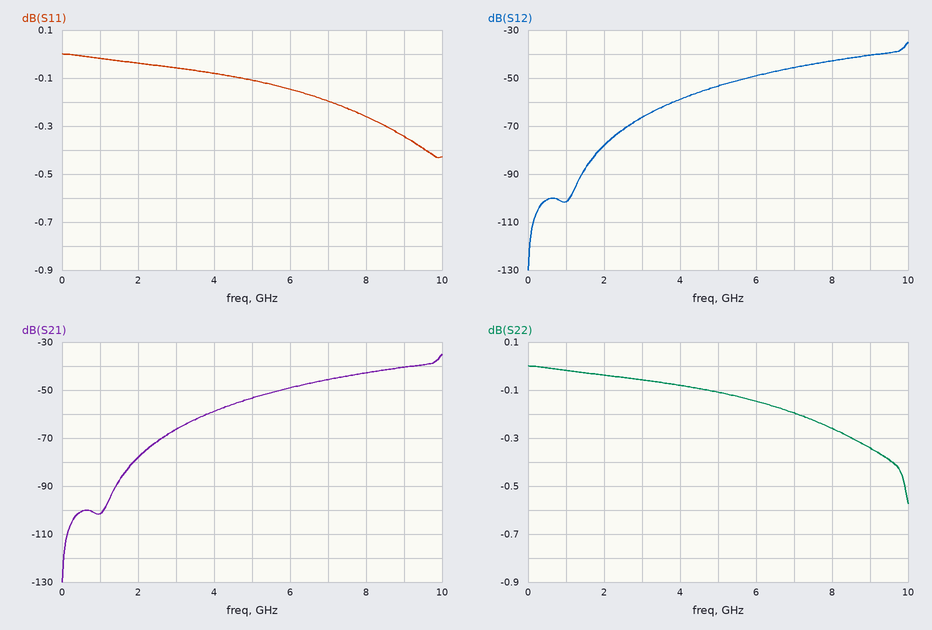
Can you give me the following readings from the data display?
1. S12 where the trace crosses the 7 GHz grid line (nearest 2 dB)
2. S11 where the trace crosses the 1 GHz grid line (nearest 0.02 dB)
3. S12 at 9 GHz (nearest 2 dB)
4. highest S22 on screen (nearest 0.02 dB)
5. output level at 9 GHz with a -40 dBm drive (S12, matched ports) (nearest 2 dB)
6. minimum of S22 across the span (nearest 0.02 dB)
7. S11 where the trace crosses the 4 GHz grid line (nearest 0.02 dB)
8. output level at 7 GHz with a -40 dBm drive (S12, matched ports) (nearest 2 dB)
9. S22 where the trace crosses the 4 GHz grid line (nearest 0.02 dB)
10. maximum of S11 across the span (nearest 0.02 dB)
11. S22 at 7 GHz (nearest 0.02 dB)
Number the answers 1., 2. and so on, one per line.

1. -46 dB
2. -0.02 dB
3. -40 dB
4. 0.00 dB
5. -80 dBm
6. -0.58 dB
7. -0.08 dB
8. -86 dBm
9. -0.08 dB
10. 0.00 dB
11. -0.20 dB
